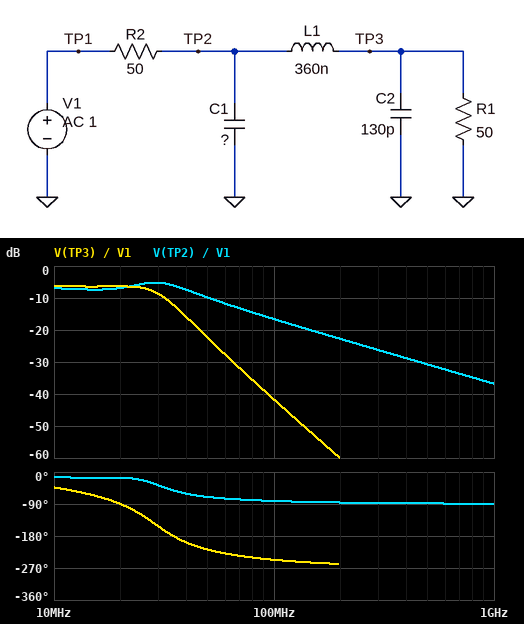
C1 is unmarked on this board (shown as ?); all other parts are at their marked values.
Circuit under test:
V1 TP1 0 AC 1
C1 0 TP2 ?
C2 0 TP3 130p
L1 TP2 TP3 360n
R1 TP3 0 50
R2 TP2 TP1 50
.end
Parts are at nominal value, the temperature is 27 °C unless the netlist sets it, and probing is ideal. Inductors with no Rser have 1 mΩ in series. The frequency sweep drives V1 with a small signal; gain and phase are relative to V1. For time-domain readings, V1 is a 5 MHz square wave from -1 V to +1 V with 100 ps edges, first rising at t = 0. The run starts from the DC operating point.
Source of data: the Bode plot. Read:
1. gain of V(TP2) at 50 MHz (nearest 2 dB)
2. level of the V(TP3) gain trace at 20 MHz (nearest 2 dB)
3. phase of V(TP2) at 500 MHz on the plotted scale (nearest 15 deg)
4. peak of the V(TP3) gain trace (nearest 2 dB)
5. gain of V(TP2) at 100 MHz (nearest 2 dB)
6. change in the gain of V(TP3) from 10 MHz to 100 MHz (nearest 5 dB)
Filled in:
-10 dB
-6 dB
-90 deg
-6 dB
-16 dB
-35 dB
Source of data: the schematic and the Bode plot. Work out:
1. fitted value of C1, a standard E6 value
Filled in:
220 pF
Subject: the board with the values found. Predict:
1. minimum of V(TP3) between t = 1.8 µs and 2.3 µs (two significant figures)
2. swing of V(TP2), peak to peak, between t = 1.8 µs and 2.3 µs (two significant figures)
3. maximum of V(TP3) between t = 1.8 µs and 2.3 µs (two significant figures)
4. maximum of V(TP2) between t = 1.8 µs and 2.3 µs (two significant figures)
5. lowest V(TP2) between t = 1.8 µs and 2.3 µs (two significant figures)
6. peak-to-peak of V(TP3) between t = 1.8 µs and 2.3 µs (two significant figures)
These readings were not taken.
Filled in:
-580 mV
1.0 V
580 mV
520 mV
-520 mV
1.2 V
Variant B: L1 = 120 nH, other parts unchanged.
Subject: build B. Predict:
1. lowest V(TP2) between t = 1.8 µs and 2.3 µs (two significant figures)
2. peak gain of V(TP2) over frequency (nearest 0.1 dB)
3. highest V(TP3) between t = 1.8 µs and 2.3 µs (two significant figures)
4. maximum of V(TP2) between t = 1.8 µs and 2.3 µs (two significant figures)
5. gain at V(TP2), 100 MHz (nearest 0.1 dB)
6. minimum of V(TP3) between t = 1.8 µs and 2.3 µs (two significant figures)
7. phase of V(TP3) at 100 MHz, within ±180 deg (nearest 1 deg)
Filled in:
-510 mV
-6.0 dB
520 mV
510 mV
-15.9 dB
-520 mV
116 deg
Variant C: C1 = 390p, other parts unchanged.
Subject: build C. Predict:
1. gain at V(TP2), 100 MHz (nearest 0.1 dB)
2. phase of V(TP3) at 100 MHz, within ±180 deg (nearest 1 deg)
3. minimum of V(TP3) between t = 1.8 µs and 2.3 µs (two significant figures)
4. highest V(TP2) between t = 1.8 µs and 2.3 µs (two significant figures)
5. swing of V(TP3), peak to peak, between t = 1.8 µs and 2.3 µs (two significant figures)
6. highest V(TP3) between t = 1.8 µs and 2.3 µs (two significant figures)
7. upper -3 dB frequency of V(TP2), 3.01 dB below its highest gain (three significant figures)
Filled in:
-21.6 dB
109 deg
-510 mV
500 mV
1.0 V
510 mV
27.1 MHz
